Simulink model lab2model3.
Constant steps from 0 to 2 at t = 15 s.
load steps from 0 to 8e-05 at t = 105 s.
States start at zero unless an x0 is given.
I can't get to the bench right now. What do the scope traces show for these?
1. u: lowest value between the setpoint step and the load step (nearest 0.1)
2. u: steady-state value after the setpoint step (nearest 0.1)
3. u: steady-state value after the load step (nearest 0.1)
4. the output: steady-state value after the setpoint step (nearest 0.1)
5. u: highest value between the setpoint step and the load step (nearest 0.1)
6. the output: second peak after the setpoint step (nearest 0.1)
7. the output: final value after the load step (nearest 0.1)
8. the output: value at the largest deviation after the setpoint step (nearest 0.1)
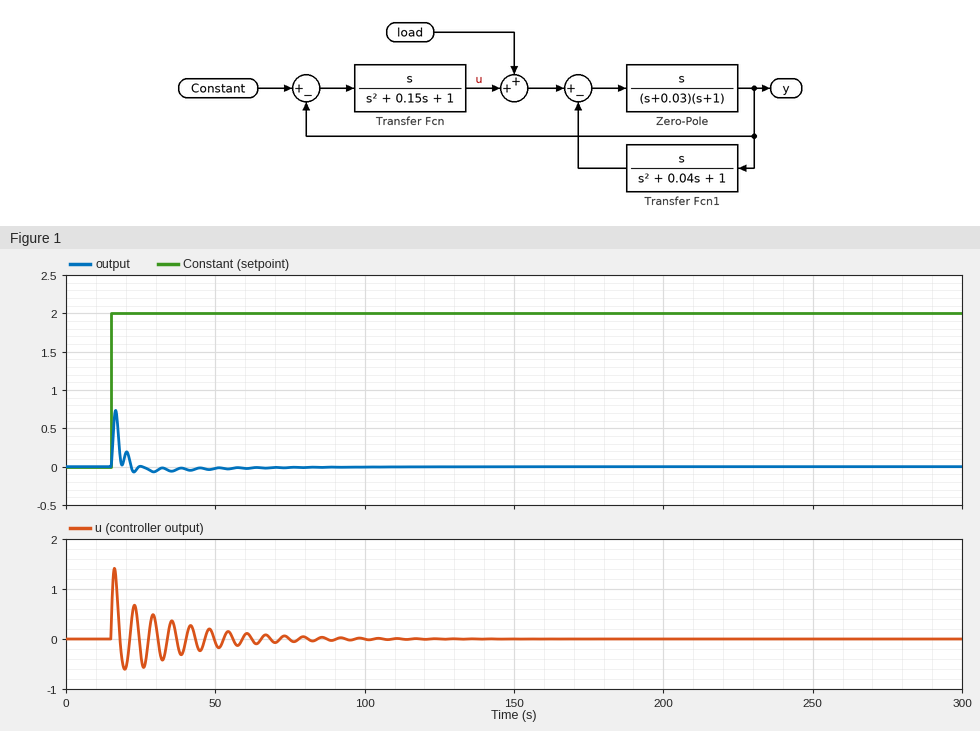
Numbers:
-0.6
0.0
0.0
0.0
1.4
0.2
0.0
0.7
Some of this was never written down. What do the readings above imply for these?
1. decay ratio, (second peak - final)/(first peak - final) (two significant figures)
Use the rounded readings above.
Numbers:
0.29
